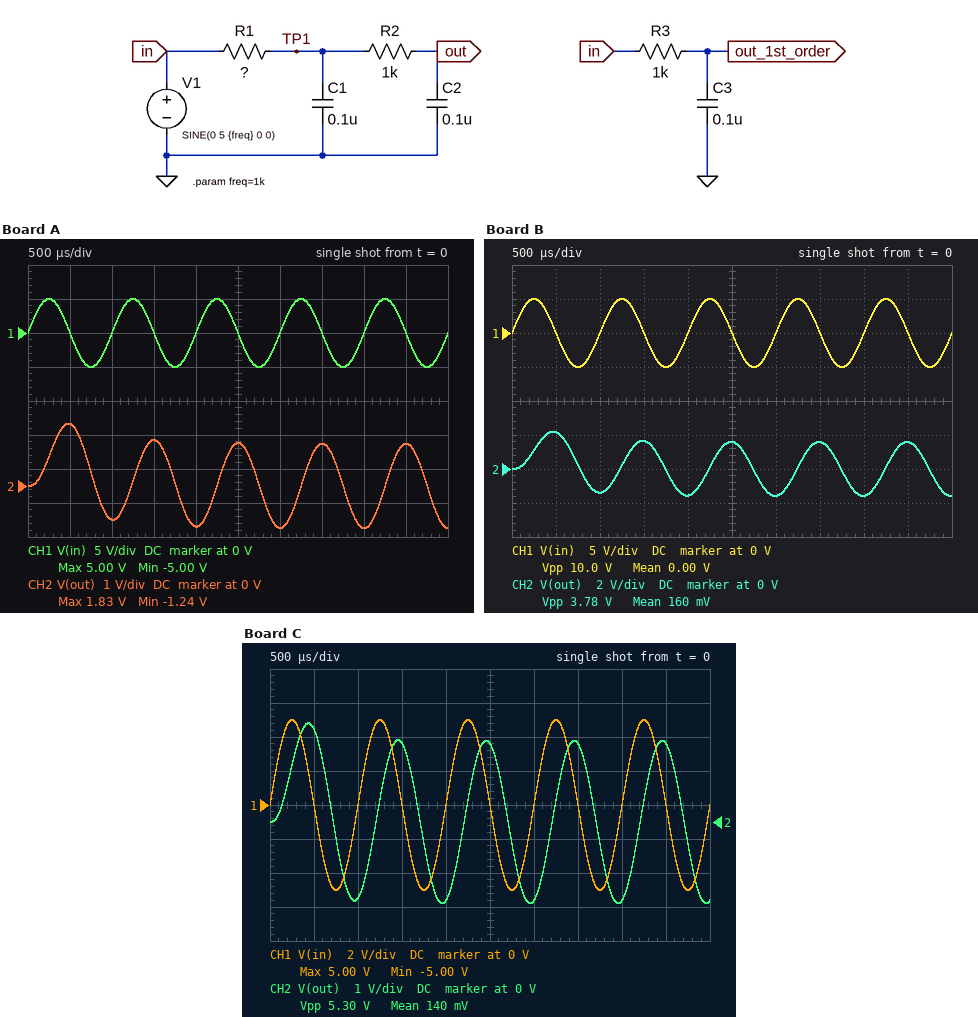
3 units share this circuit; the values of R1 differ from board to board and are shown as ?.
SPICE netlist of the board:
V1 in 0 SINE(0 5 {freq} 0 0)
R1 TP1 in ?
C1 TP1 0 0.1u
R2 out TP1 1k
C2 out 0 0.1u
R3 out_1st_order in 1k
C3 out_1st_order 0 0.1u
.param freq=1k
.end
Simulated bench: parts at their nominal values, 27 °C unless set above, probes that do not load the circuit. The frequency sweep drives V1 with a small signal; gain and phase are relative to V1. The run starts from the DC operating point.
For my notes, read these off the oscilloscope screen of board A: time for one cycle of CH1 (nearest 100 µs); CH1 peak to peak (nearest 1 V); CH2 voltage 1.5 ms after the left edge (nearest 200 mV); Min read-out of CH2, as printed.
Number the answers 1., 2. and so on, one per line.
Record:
1. 1.0 ms
2. 10 V
3. 1.4 V
4. -1.24 V
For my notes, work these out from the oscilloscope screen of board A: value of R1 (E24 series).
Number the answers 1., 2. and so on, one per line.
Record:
1. 2.7 kΩ
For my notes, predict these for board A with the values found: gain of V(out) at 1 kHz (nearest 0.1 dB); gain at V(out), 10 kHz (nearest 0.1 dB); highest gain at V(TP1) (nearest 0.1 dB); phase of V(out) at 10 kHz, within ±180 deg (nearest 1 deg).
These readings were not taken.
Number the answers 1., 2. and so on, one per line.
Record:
1. -12.1 dB
2. -41.1 dB
3. 0 dB
4. -159 deg
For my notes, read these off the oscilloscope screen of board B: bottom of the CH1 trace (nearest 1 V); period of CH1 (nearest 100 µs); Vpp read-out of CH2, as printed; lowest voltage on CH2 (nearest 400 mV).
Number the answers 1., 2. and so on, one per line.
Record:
1. -5 V
2. 1.0 ms
3. 3.78 V
4. -1.6 V
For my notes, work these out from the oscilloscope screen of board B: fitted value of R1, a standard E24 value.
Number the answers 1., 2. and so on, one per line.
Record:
1. 2 kΩ
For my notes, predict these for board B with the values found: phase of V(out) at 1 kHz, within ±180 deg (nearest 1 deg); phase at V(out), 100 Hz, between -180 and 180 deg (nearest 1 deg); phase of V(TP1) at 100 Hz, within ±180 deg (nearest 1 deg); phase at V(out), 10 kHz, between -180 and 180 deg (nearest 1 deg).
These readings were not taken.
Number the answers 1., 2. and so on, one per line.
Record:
1. -86 deg
2. -18 deg
3. -14 deg
4. -158 deg
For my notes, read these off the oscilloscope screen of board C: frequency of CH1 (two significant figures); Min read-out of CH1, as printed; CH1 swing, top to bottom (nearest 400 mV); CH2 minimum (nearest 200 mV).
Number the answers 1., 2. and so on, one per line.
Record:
1. 1.0 kHz
2. -5.00 V
3. 10.0 V
4. -2.4 V
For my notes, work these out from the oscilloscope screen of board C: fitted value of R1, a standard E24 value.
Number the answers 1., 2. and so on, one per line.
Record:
1. 1.1 kΩ
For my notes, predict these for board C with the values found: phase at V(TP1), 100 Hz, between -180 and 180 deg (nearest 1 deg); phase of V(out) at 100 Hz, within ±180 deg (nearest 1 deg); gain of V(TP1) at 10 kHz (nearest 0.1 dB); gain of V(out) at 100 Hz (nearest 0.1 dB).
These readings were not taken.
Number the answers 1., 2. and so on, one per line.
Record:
1. -8 deg
2. -11 deg
3. -17.4 dB
4. -0.1 dB
